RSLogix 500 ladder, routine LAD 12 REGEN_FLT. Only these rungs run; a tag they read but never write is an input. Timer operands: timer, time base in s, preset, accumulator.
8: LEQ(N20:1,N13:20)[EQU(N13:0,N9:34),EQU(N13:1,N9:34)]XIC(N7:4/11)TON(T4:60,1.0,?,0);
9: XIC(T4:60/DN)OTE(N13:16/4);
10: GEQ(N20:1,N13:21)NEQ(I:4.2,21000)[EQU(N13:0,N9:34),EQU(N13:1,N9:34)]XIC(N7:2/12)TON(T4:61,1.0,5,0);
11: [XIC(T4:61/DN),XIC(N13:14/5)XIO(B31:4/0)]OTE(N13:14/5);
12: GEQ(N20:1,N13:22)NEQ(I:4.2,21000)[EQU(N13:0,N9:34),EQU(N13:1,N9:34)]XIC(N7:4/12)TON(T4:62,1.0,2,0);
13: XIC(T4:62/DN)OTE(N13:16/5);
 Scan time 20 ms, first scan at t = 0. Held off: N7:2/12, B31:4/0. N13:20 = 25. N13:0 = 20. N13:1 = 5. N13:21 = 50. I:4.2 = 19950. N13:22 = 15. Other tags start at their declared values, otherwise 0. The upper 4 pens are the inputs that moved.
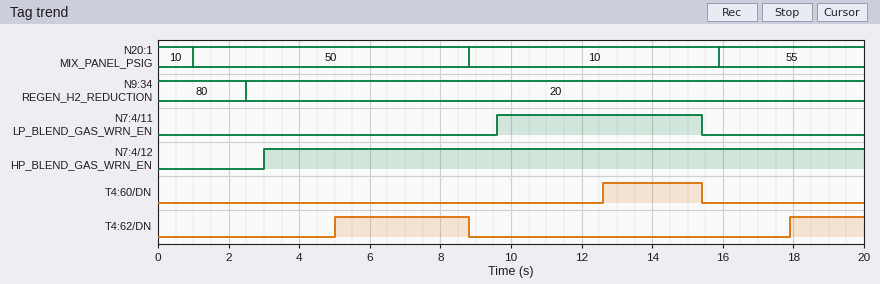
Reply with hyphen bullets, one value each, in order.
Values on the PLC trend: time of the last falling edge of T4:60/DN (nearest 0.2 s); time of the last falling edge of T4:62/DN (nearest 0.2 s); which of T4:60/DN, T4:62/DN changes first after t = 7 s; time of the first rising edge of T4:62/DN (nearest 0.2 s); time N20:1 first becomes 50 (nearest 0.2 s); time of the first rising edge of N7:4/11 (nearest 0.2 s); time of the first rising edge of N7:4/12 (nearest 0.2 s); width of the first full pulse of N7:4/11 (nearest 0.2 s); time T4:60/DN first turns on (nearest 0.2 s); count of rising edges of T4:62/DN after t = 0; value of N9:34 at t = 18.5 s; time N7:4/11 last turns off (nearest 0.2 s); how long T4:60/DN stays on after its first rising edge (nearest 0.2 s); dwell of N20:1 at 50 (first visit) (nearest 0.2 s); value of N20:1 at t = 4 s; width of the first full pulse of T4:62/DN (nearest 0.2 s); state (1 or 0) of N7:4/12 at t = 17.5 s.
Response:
- 15.4 s
- 8.8 s
- T4:62/DN
- 5.0 s
- 1.0 s
- 9.6 s
- 3.0 s
- 5.8 s
- 12.6 s
- 2
- 20
- 15.4 s
- 2.8 s
- 7.8 s
- 50
- 3.8 s
- 1
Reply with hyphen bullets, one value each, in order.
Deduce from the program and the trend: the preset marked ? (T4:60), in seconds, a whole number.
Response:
- 3 s
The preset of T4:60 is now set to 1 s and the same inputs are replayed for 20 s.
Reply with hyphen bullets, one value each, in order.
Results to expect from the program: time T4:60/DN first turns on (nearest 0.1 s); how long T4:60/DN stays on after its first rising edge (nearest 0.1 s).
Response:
- 10.6 s
- 4.8 s
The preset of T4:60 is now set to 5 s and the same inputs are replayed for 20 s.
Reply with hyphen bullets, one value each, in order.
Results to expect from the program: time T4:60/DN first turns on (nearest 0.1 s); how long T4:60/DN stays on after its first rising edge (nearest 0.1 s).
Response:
- 14.6 s
- 0.8 s
